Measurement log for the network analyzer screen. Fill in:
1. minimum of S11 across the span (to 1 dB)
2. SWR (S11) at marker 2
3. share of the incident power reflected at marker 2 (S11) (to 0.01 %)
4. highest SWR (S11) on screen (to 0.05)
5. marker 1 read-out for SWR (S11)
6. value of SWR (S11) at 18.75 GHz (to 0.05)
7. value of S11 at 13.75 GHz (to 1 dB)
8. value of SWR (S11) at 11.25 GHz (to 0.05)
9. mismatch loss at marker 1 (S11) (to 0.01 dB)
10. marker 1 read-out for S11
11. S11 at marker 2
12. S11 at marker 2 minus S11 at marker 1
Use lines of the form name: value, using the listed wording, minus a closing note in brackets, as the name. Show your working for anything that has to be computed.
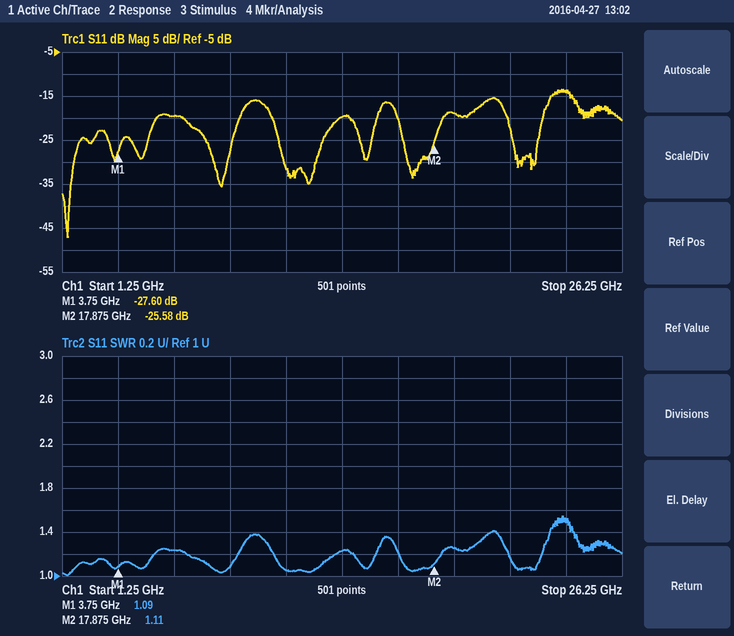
minimum of S11 across the span: -47 dB
SWR (S11) at marker 2: 1.11
share of the incident power reflected at marker 2 (S11): 10^(-25.58/10) ≈ 0.28 %
highest SWR (S11) on screen: 1.55
marker 1 read-out for SWR: 1.09
value of SWR (S11) at 18.75 GHz: 1.25
value of S11 at 13.75 GHz: -20 dB
value of SWR (S11) at 11.25 GHz: 1.05
mismatch loss at marker 1 (S11): −10 log10(1 − 10^(-27.6/10)) ≈ 0.01 dB
marker 1 read-out for S11: -27.60 dB
S11 at marker 2: -25.58 dB
S11 at marker 2 minus S11 at marker 1: -25.58 − (-27.6) = 2.02 dB
